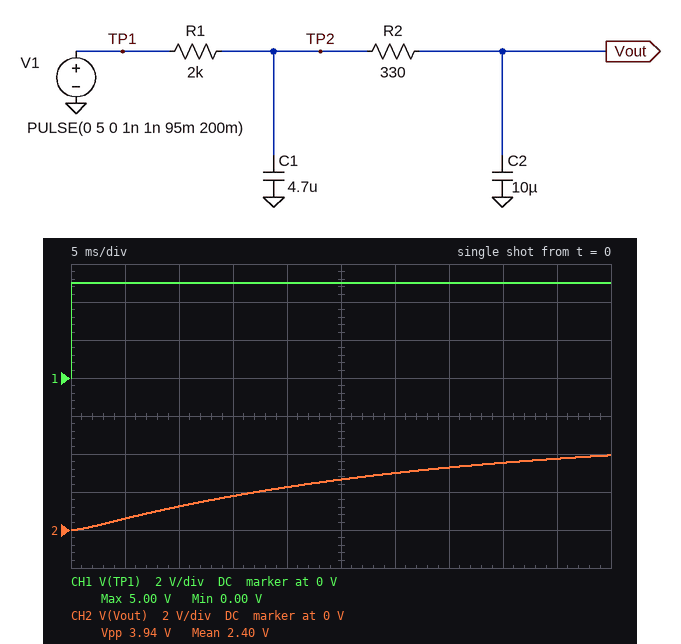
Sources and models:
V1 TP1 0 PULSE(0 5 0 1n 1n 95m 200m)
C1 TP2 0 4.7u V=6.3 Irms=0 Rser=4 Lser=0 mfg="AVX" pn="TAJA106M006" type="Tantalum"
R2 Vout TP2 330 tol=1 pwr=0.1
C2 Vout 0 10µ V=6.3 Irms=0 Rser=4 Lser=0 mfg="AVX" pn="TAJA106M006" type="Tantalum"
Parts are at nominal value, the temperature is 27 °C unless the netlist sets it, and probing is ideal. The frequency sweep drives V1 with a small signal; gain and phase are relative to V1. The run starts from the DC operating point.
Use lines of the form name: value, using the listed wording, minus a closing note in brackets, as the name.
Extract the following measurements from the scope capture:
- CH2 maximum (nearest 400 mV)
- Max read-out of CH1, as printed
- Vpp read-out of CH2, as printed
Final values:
CH2 maximum: 4.0 V
Max read-out of CH1, as printed: 5.00 V
Vpp read-out of CH2, as printed: 3.94 V
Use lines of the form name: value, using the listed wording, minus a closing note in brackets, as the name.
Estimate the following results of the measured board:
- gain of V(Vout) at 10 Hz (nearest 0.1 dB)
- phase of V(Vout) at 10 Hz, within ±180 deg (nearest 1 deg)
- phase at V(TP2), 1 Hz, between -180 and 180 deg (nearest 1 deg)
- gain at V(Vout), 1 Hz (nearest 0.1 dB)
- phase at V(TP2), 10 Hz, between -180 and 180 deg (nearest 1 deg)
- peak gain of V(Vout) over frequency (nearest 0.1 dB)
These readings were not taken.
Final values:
gain of V(Vout) at 10 Hz: -7.0 dB
phase of V(Vout) at 10 Hz, within ±180 deg: -67 deg
phase at V(TP2), 1 Hz, between -180 and 180 deg: -10 deg
gain at V(Vout), 1 Hz: -0.2 dB
phase at V(TP2), 10 Hz, between -180 and 180 deg: -55 deg
peak gain of V(Vout) over frequency: 0 dB
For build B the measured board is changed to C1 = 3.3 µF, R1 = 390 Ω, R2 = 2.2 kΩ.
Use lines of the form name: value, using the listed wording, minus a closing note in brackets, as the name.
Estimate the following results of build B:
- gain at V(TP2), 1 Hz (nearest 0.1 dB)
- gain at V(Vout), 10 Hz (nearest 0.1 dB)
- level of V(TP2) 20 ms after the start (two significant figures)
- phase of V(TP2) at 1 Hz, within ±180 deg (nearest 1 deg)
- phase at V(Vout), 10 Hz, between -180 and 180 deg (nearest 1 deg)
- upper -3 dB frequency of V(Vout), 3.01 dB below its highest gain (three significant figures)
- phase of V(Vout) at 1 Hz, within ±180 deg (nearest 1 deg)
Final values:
gain at V(TP2), 1 Hz: 0 dB
gain at V(Vout), 10 Hz: -5.7 dB
level of V(TP2) 20 ms after the start: 4.6 V
phase of V(TP2) at 1 Hz, within ±180 deg: -2 deg
phase at V(Vout), 10 Hz, between -180 and 180 deg: -62 deg
upper -3 dB frequency of V(Vout), 3.01 dB below its highest gain: 6.08 Hz
phase of V(Vout) at 1 Hz, within ±180 deg: -10 deg
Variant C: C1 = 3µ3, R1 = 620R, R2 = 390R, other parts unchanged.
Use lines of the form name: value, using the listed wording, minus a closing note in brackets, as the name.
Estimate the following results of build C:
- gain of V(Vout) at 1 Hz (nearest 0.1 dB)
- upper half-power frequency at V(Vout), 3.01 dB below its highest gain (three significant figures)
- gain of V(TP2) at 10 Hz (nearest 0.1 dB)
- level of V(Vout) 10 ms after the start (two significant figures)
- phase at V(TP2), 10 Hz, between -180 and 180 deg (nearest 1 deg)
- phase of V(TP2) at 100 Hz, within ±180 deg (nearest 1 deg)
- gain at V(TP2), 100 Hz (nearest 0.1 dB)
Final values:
gain of V(Vout) at 1 Hz: 0 dB
upper half-power frequency at V(Vout), 3.01 dB below its highest gain: 13.8 Hz
gain of V(TP2) at 10 Hz: -1.6 dB
level of V(Vout) 10 ms after the start: 2.8 V
phase at V(TP2), 10 Hz, between -180 and 180 deg: -24 deg
phase of V(TP2) at 100 Hz, within ±180 deg: -38 deg
gain at V(TP2), 100 Hz: -9.5 dB
